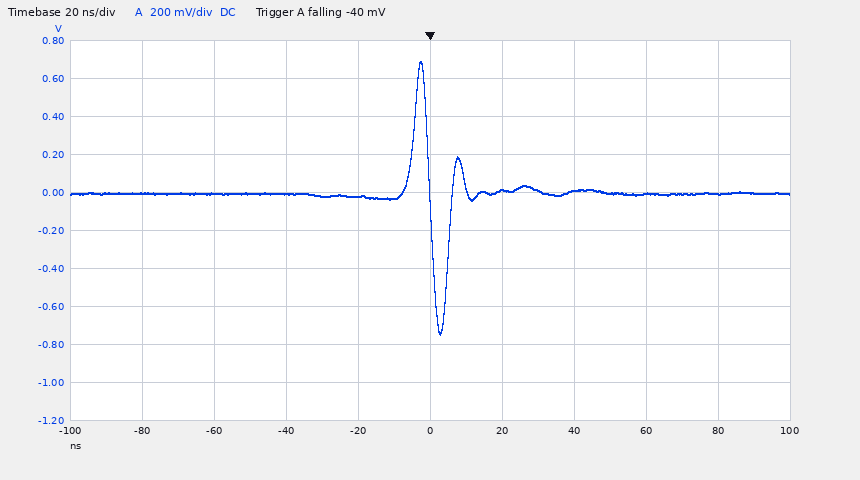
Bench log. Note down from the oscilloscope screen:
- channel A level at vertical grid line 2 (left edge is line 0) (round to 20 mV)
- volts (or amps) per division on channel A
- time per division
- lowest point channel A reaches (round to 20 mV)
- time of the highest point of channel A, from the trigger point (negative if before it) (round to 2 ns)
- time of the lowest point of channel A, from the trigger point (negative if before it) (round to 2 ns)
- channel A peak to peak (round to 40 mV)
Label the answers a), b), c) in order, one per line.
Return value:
a) 0 mV
b) 200 mV
c) 20 ns
d) -740 mV
e) -2 ns
f) +2 ns
g) 1.44 V
